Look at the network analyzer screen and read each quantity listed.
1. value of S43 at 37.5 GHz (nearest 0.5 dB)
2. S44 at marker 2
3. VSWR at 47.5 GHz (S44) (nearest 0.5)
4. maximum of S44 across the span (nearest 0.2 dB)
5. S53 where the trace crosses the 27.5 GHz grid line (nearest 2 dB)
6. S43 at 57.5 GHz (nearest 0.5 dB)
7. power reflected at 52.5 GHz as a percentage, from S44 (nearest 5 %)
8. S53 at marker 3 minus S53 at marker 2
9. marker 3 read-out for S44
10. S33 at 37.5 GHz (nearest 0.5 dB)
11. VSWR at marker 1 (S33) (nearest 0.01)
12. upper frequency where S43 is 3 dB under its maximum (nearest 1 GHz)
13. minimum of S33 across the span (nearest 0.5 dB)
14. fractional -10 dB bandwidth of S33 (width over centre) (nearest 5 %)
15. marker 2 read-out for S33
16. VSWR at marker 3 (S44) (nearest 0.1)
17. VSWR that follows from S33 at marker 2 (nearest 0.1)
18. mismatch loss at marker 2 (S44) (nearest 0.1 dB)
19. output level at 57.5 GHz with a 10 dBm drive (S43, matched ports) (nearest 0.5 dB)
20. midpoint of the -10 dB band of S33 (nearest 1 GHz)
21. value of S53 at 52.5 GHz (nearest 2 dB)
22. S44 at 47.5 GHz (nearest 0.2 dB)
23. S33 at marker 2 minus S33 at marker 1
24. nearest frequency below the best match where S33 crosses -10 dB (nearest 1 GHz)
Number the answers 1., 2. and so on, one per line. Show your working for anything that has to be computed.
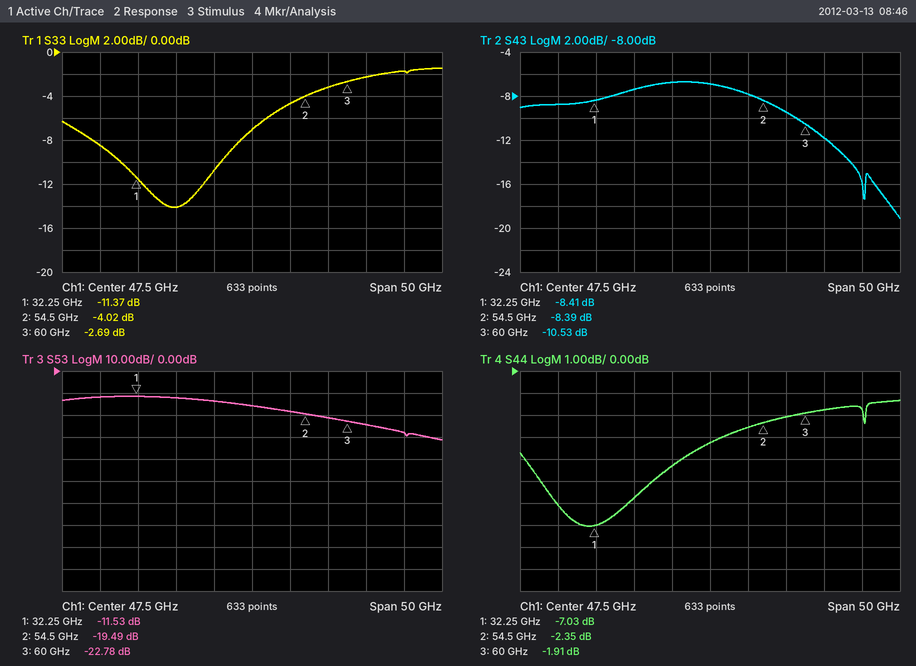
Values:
1. -7.5 dB
2. -2.35 dB
3. |Γ| = 10^(-3.2/20) = 0.6918; VSWR = (1 + 0.6918)/(1 − 0.6918) ≈ 5.5
4. -1.4 dB
5. -12 dB
6. -9.5 dB
7. 10^(-2.6/10) ≈ 55 %
8. -22.78 − (-19.49) = -3.29 dB
9. -1.91 dB
10. -14.0 dB
11. (1 + 0.2701)/(1 − 0.2701) ≈ 1.74
12. 58 GHz
13. -14.0 dB
14. 13 GHz / 36.5 GHz ≈ 35.6 %, so 35 % to the nearest 5 %
15. -4.02 dB
16. (1 + 0.8026)/(1 − 0.8026) ≈ 9.1
17. (1 + 0.6295)/(1 − 0.6295) ≈ 4.4
18. −10 log10(1 − 10^(-2.35/10)) ≈ 3.8 dB
19. 10 dBm + (-9.5 dB) = 0.5 dBm
20. 37 GHz
21. -18 dB
22. -3.2 dB
23. -4.02 − (-11.37) = 7.35 dB
24. 30 GHz
